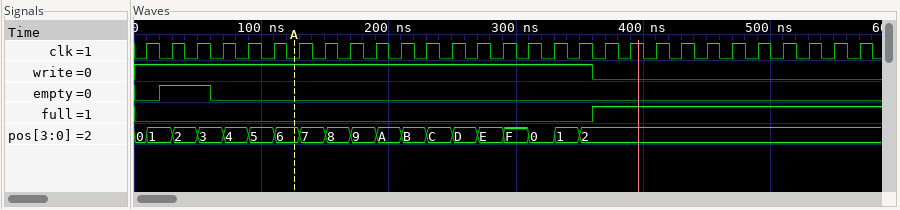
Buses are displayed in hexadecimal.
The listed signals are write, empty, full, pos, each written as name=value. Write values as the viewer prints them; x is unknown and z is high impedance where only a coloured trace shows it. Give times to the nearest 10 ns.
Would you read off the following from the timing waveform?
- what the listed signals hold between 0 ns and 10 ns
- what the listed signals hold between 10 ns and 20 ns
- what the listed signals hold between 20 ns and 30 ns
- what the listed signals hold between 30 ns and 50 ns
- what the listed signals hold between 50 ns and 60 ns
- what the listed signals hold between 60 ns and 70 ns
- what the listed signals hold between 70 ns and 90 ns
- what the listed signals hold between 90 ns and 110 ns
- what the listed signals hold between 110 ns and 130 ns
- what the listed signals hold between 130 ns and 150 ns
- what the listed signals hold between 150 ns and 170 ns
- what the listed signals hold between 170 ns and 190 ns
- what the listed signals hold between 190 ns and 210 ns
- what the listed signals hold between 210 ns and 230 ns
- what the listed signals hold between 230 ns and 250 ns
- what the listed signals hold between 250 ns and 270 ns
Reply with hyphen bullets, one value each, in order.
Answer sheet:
- write=1, empty=0, full=0, pos=0
- write=1, empty=0, full=0, pos=1
- write=1, empty=1, full=0, pos=1
- write=1, empty=1, full=0, pos=2
- write=1, empty=1, full=0, pos=3
- write=1, empty=0, full=0, pos=3
- write=1, empty=0, full=0, pos=4
- write=1, empty=0, full=0, pos=5
- write=1, empty=0, full=0, pos=6
- write=1, empty=0, full=0, pos=7
- write=1, empty=0, full=0, pos=8
- write=1, empty=0, full=0, pos=9
- write=1, empty=0, full=0, pos=A
- write=1, empty=0, full=0, pos=B
- write=1, empty=0, full=0, pos=C
- write=1, empty=0, full=0, pos=D
